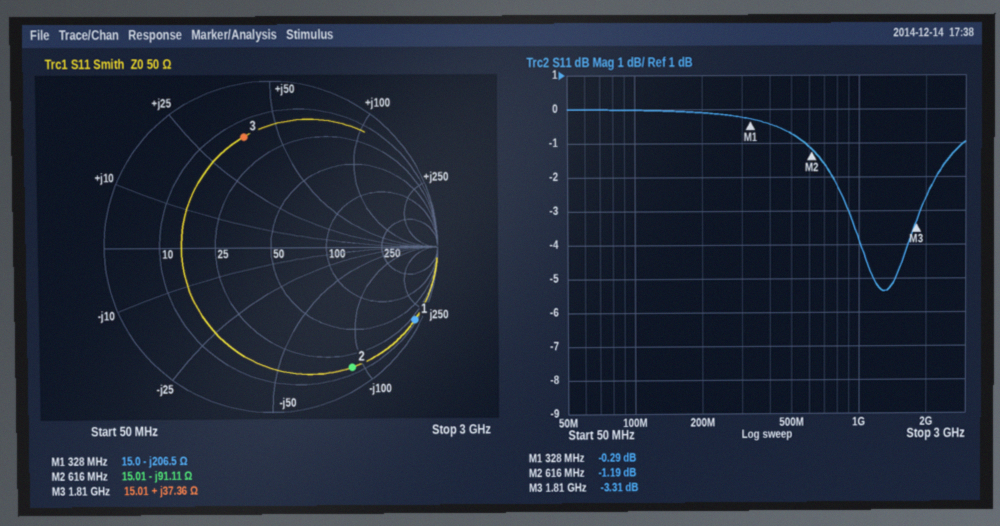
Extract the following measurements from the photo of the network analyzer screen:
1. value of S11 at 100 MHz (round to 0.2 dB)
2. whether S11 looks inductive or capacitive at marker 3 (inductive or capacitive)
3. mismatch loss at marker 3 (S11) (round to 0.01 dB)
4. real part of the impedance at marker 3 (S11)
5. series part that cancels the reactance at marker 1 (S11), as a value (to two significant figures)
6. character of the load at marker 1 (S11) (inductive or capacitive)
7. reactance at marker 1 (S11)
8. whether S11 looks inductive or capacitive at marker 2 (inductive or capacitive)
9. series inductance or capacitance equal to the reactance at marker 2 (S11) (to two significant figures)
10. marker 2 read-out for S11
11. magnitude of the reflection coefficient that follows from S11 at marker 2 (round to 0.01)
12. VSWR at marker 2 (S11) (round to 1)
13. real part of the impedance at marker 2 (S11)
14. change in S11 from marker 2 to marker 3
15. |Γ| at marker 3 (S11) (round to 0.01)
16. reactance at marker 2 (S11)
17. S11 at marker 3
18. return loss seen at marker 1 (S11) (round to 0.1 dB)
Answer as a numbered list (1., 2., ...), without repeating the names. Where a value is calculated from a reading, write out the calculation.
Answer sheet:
1. 0.0 dB
2. inductive
3. −10 log10(1 − 10^(-3.31/10)) ≈ 2.73 dB
4. 15.01 Ω
5. L = 206.5 Ω/(2π × 328 MHz) ≈ 100 nH
6. capacitive
7. -206.5 Ω
8. capacitive
9. C = 1/(2π × 616 MHz × 91.11 Ω) ≈ 2.8 pF
10. -1.19 dB
11. 10^(-1.19/20) ≈ 0.87
12. 15
13. 15.01 Ω
14. -3.31 − (-1.19) = -2.12 dB
15. 0.68
16. -91.11 Ω
17. -3.31 dB
18. 0.3 dB
